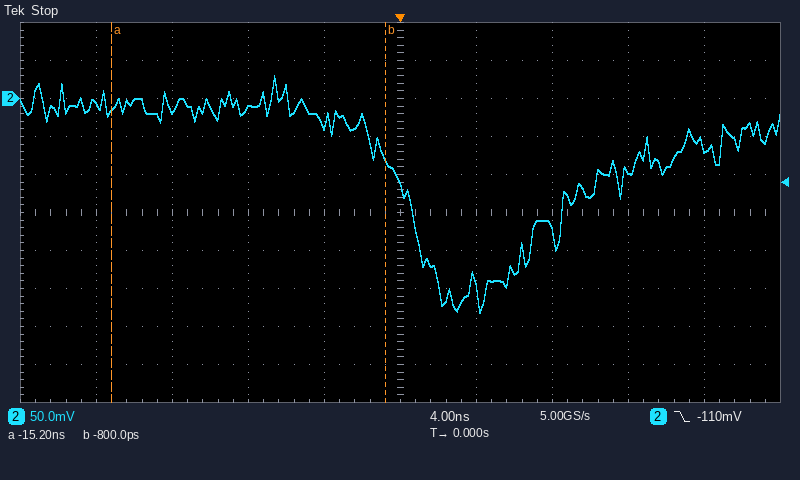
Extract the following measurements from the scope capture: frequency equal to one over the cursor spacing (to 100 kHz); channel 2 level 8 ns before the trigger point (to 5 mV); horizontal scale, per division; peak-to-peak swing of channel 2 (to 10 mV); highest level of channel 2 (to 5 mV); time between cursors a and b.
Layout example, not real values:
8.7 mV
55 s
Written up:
69.4 MHz
-15 mV
4 ns
310 mV
30 mV
14.4 ns
